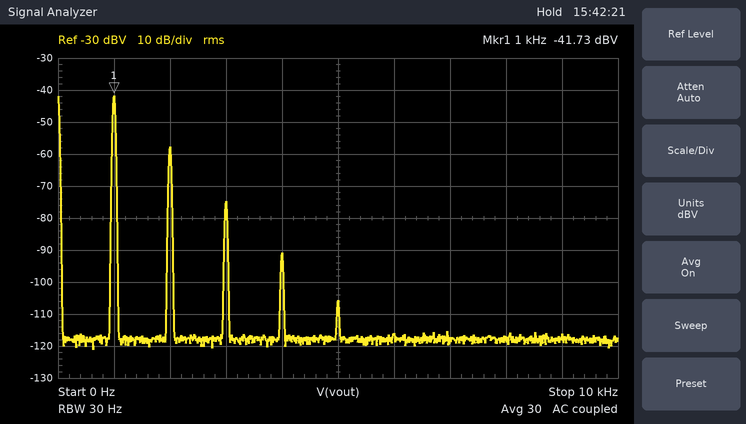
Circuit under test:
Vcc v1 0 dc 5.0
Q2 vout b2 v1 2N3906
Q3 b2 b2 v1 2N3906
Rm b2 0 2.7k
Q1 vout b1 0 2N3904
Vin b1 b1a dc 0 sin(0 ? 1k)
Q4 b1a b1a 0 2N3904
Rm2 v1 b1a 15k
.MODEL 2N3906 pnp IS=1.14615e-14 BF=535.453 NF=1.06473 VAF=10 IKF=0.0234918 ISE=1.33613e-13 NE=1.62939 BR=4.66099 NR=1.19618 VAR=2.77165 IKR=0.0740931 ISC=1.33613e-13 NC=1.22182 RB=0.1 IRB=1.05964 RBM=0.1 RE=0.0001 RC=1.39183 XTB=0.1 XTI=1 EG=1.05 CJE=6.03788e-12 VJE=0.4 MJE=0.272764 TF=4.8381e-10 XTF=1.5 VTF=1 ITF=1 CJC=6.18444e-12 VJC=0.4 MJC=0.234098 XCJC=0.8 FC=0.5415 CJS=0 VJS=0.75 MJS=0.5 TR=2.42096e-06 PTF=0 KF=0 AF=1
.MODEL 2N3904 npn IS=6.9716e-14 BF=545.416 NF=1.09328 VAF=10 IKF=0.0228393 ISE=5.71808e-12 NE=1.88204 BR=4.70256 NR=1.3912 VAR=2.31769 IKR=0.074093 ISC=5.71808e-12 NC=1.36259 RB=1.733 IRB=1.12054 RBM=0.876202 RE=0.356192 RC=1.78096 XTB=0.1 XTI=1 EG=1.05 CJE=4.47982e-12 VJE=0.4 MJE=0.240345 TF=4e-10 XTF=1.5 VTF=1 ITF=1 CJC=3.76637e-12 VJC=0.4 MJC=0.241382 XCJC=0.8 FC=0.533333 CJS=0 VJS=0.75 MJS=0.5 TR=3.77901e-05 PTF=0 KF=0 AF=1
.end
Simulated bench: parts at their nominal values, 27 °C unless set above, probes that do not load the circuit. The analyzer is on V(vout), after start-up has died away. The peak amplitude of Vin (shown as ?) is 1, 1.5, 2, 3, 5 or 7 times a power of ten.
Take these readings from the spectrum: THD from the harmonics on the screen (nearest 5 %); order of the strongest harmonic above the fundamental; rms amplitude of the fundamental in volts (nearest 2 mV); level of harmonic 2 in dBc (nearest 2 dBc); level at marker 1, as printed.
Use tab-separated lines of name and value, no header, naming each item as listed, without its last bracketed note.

THD from the harmonics on the screen	15 %
order of the strongest harmonic above the fundamental	2
rms amplitude of the fundamental in volts	8 mV
level of harmonic 2 in dBc	-16 dBc
level at marker 1, as printed	-41.73 dBV
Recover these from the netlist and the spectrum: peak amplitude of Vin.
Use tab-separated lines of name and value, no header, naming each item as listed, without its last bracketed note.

peak amplitude of Vin	15 mV
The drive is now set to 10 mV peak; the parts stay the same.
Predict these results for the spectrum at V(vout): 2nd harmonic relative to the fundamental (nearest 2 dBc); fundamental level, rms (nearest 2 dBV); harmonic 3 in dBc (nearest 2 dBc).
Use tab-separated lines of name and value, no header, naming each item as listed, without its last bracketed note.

2nd harmonic relative to the fundamental	-20 dBc
fundamental level, rms	-46 dBV
harmonic 3 in dBc	-40 dBc
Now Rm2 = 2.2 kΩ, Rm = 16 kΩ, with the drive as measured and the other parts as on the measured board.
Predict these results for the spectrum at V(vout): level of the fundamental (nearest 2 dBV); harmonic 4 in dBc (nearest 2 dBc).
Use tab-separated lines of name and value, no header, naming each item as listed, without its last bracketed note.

level of the fundamental	-46 dBV
harmonic 4 in dBc	-52 dBc
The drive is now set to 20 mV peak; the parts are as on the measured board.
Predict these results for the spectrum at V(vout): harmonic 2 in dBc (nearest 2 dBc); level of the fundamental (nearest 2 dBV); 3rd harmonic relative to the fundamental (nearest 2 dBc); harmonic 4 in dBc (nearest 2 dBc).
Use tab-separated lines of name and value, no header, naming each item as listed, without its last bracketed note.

harmonic 2 in dBc	-14 dBc
level of the fundamental	-38 dBV
3rd harmonic relative to the fundamental	-28 dBc
harmonic 4 in dBc	-40 dBc
